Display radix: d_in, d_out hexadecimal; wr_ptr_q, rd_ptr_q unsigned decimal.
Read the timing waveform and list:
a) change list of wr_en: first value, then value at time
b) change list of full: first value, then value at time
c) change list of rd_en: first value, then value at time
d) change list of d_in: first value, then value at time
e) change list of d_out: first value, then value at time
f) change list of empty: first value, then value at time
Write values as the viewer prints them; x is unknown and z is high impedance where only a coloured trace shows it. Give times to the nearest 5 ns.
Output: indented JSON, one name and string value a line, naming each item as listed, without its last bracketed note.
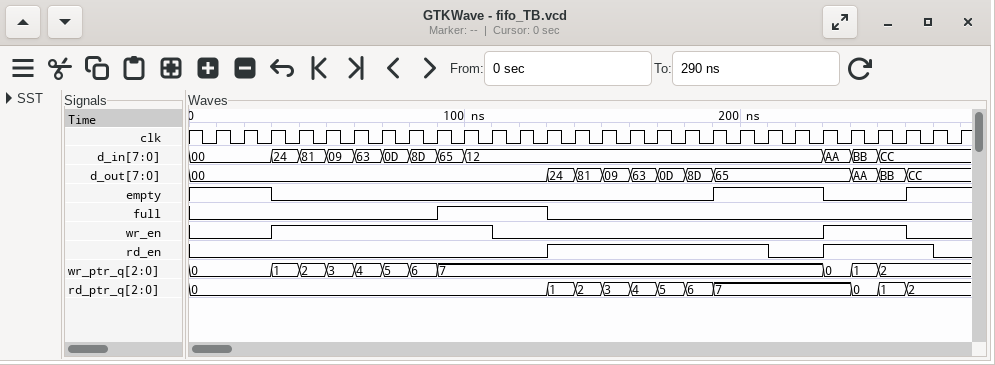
{
  "change list of wr_en: first value, then value at time": "0, 1 at 30 ns, 0 at 110 ns, 1 at 230 ns, 0 at 260 ns",
  "change list of full: first value, then value at time": "0, 1 at 90 ns, 0 at 130 ns",
  "change list of rd_en: first value, then value at time": "0, 1 at 130 ns, 0 at 210 ns, 1 at 230 ns, 0 at 270 ns",
  "change list of d_in: first value, then value at time": "00, 24 at 30 ns, 81 at 40 ns, 09 at 50 ns, 63 at 60 ns, 0D at 70 ns, 8D at 80 ns, 65 at 90 ns, 12 at 100 ns, AA at 230 ns, BB at 240 ns, CC at 250 ns",
  "change list of d_out: first value, then value at time": "00, 24 at 130 ns, 81 at 140 ns, 09 at 150 ns, 63 at 160 ns, 0D at 170 ns, 8D at 180 ns, 65 at 190 ns, AA at 240 ns, BB at 250 ns, CC at 260 ns",
  "change list of empty: first value, then value at time": "1, 0 at 30 ns, 1 at 190 ns, 0 at 230 ns, 1 at 260 ns"
}
